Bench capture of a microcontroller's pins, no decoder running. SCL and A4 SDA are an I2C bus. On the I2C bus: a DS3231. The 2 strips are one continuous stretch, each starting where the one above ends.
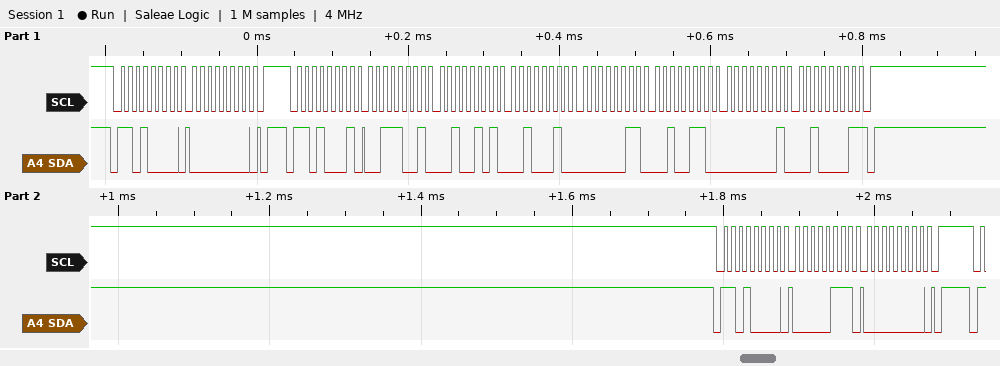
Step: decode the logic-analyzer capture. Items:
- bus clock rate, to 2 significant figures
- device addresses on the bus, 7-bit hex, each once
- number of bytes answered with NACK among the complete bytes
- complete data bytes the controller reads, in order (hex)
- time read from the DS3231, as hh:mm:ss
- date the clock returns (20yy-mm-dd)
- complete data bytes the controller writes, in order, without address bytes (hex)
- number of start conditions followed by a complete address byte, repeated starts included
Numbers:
100 kHz
0x68
1
39 25 22 03 26 01 21
22:25:39
2021-01-26
00 07 00
3
